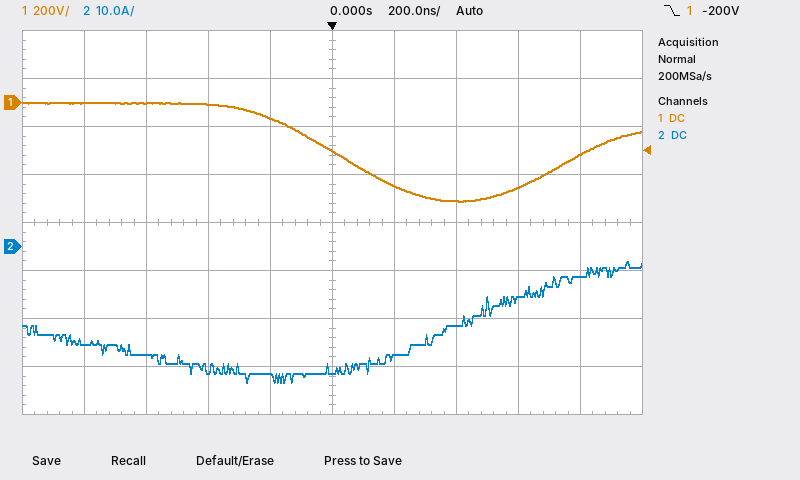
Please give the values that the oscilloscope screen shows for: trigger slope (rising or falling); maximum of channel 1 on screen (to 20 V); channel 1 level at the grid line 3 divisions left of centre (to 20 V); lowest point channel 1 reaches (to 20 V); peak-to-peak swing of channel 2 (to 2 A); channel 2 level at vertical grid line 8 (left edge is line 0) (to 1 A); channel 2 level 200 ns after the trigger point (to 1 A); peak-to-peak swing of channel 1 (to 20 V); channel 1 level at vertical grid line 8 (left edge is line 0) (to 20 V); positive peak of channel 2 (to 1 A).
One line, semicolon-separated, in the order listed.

falling; 0 V; 0 V; -420 V; 26 A; -11 A; -23 A; 420 V; -360 V; -3 A
